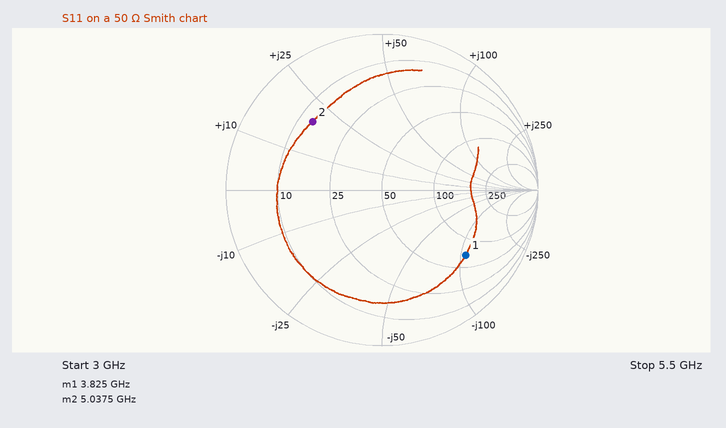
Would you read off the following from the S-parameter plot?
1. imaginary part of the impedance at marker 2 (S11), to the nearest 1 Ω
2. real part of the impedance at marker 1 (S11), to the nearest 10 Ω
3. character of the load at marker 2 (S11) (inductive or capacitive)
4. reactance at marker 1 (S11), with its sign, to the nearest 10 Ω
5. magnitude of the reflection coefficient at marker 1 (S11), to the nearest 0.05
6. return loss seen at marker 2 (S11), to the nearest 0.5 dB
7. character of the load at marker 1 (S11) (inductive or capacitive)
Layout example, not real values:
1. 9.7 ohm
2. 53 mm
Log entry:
1. +19 Ω
2. 70 Ω
3. inductive
4. -110 Ω
5. 0.70
6. 4.0 dB
7. capacitive
